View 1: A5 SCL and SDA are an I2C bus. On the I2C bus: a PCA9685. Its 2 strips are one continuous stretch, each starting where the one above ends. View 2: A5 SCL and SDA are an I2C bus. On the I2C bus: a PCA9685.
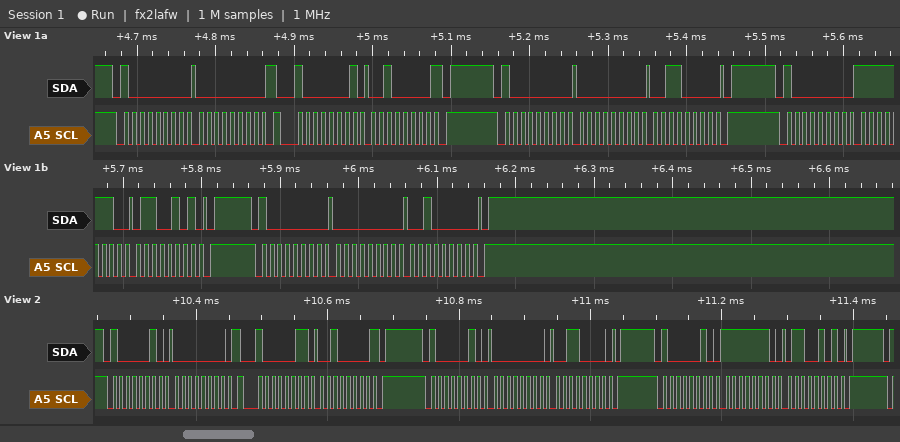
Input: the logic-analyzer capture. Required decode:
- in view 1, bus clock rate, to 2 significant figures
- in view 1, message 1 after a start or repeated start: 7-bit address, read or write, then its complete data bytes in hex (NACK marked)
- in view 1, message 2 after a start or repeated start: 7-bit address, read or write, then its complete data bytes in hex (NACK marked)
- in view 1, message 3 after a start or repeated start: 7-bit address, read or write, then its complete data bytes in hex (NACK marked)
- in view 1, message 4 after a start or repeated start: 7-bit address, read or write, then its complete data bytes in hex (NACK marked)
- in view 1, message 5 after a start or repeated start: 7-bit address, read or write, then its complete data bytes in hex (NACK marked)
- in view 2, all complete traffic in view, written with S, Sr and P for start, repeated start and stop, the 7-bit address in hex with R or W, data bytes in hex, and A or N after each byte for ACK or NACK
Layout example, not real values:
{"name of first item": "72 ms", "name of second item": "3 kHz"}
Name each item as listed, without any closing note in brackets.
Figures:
{"in view 1, bus clock rate, to 2 significant figures": "100 kHz", "in view 1, message 1 after a start or repeated start: 7-bit address, read or write, then its complete data bytes in hex": "0x40 write: 00", "in view 1, message 2 after a start or repeated start: 7-bit address, read or write, then its complete data bytes in hex": "0x40 read: 20 NACK", "in view 1, message 3 after a start or repeated start: 7-bit address, read or write, then its complete data bytes in hex": "0x40 write: 00 30", "in view 1, message 4 after a start or repeated start: 7-bit address, read or write, then its complete data bytes in hex": "0x40 write: FE 65", "in view 1, message 5 after a start or repeated start: 7-bit address, read or write, then its complete data bytes in hex": "0x40 write: 00 20", "in view 2, all complete traffic in view, written with S, Sr and P for start, repeated start and stop, the 7-bit address in hex with R or W, data bytes in hex, and A or N after each byte for ACK or NACK": "S 41W A 00 A Sr 41R A 20 N P S 41W A 00 A 30 A P S 41W A FE A 65 A P"}
